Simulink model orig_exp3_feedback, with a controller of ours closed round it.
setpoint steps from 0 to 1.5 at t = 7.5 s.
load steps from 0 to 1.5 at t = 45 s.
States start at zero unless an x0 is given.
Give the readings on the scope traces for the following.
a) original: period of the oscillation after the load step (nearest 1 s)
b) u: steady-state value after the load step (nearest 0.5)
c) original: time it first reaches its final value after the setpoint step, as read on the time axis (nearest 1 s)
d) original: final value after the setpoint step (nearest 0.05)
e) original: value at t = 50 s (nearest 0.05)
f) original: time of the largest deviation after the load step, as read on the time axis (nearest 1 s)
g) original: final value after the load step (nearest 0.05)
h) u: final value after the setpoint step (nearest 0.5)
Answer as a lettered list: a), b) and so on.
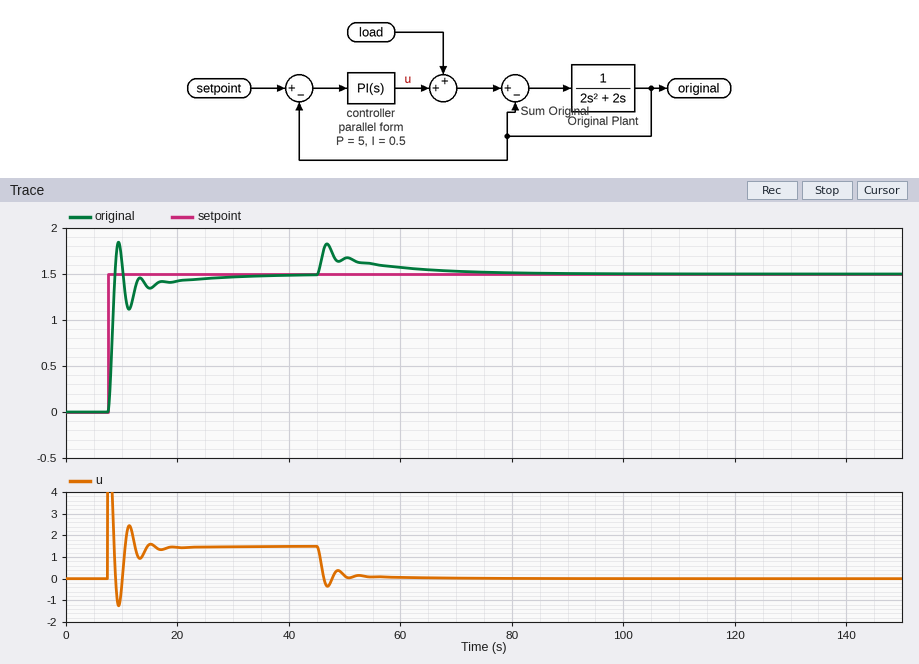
a) 4 s
b) 0.0
c) 9 s
d) 1.50
e) 1.65
f) 47 s
g) 1.50
h) 1.5
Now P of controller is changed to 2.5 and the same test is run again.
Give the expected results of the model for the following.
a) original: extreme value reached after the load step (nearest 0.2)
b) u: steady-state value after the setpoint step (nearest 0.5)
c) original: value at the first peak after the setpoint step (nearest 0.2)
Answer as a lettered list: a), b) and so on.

a) 2.0
b) 1.5
c) 1.6
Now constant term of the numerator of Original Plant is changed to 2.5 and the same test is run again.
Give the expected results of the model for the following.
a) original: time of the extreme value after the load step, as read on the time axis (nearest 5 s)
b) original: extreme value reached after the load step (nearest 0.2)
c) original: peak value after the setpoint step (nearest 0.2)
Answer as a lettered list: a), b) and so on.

a) 45 s
b) 1.8
c) 2.0
